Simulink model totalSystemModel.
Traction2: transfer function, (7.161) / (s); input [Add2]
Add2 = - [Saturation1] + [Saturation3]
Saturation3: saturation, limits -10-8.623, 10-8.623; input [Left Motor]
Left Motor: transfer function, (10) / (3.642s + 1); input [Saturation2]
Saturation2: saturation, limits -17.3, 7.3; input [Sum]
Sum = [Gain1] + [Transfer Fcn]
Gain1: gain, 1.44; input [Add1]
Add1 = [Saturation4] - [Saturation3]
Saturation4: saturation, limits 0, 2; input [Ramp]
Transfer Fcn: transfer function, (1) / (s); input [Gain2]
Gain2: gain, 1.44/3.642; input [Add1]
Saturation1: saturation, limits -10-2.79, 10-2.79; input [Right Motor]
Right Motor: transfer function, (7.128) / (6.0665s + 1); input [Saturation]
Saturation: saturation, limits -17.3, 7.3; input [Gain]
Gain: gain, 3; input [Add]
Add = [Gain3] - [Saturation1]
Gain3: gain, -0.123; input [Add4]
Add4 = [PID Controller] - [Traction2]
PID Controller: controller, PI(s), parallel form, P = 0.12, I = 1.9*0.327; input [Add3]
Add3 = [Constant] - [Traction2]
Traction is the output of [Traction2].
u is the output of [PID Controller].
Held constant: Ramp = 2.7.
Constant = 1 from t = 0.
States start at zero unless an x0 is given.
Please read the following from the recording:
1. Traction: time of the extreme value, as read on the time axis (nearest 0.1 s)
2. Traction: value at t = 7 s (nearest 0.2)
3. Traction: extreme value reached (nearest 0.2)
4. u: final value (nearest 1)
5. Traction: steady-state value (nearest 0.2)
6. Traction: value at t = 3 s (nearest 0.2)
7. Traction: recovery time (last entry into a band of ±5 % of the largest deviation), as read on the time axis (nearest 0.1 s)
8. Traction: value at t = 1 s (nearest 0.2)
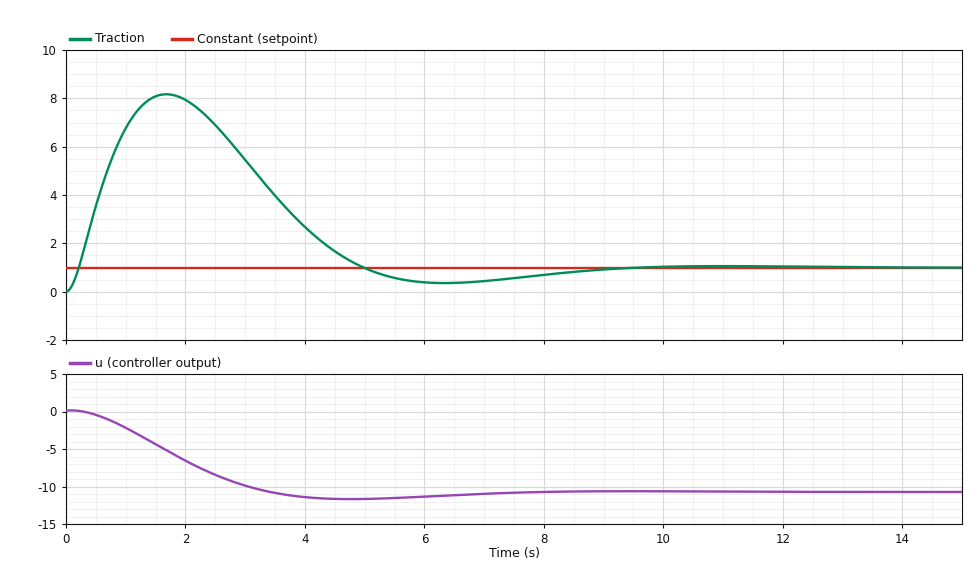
1.7 s
0.4
8.2
-11
1.0
5.4
7.6 s
6.8
